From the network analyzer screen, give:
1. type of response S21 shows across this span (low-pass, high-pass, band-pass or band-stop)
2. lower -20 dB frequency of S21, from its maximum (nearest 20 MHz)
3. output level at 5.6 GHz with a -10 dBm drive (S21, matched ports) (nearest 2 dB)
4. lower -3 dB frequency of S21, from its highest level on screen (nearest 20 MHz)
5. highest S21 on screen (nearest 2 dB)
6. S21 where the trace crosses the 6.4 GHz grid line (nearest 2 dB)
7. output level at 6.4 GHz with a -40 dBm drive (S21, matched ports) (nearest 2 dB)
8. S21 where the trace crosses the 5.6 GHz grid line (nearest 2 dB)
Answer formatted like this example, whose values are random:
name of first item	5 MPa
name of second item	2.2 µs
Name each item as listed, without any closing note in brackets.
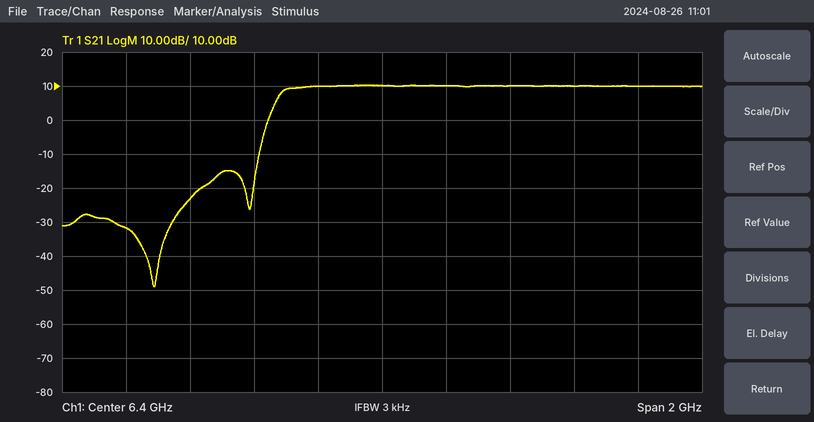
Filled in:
type of response S21 shows across this span	high-pass
lower -20 dB frequency of S21, from its maximum	6.02 GHz
output level at 5.6 GHz with a -10 dBm drive (S21, matched ports)	-42 dBm
lower -3 dB frequency of S21, from its highest level on screen	6.08 GHz
highest S21 on screen	10 dB
S21 where the trace crosses the 6.4 GHz grid line	10 dB
output level at 6.4 GHz with a -40 dBm drive (S21, matched ports)	-30 dBm
S21 where the trace crosses the 5.6 GHz grid line	-32 dB
